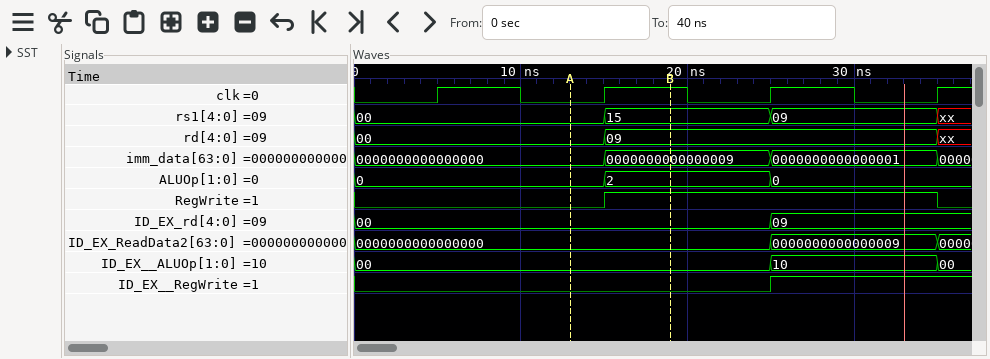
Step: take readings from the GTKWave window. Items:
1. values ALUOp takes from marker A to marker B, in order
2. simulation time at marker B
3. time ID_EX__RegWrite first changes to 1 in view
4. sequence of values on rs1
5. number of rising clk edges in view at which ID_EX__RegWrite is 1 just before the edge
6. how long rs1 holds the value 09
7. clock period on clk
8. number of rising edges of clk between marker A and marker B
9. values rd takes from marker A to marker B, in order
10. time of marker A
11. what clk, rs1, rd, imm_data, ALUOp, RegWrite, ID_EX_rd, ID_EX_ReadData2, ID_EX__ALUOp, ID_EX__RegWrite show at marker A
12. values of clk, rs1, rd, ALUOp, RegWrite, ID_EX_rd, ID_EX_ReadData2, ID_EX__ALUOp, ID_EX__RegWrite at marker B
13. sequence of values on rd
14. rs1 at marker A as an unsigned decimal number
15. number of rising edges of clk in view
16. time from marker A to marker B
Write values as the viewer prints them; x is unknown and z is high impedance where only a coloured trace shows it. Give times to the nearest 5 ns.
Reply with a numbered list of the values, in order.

1. 0, 2
2. 20 ns
3. 25 ns
4. 00, 15, 09, xx
5. 1
6. 10 ns
7. 10 ns
8. 1
9. 00, 09
10. 15 ns
11. clk=0, rs1=00, rd=00, imm_data=0000000000000000, ALUOp=0, RegWrite=0, ID_EX_rd=00, ID_EX_ReadData2=0000000000000000, ID_EX__ALUOp=00, ID_EX__RegWrite=0
12. clk=1, rs1=15, rd=09, ALUOp=2, RegWrite=1, ID_EX_rd=00, ID_EX_ReadData2=0000000000000000, ID_EX__ALUOp=00, ID_EX__RegWrite=0
13. 00, 09, xx
14. 0
15. 4
16. 5 ns
